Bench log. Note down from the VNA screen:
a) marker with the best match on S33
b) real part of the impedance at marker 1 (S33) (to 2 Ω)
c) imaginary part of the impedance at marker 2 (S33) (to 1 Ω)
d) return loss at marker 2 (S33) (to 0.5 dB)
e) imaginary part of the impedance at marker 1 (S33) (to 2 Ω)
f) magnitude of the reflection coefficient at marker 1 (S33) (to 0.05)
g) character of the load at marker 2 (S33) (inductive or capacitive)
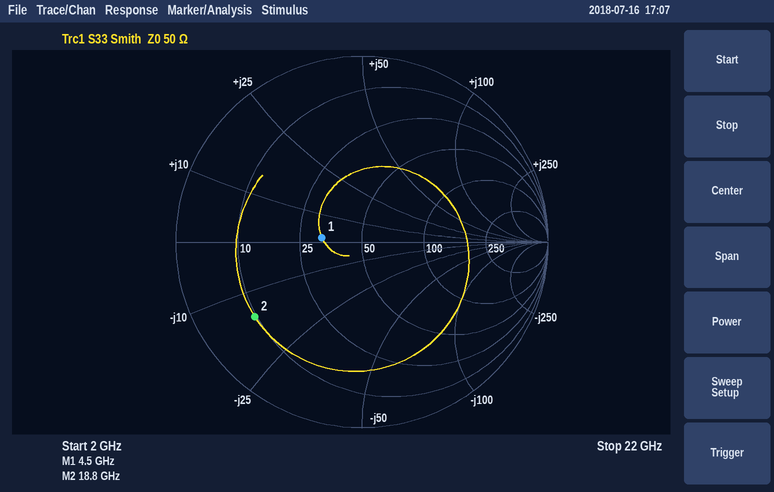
marker 1
32 Ω
-15 Ω
3.0 dB
+2 Ω
0.20
capacitive
